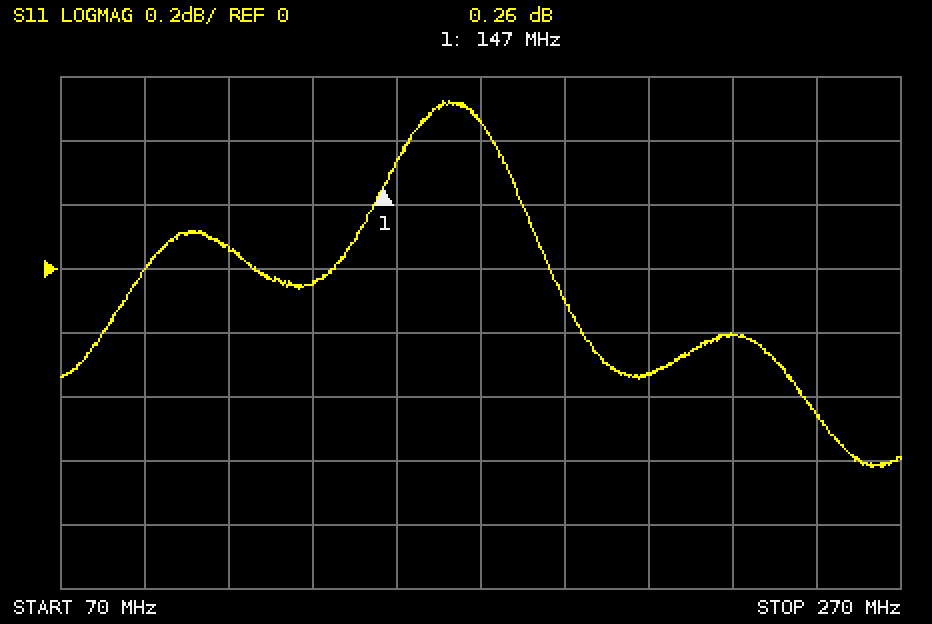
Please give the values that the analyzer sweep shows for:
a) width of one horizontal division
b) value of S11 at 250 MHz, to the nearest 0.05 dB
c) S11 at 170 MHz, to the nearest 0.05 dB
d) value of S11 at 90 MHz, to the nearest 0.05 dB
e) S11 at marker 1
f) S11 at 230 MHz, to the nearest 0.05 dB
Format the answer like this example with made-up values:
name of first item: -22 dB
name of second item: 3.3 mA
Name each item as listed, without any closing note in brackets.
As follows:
width of one horizontal division: 20 MHz
value of S11 at 250 MHz, to the nearest 0.05 dB: -0.45 dB
S11 at 170 MHz, to the nearest 0.05 dB: 0.45 dB
value of S11 at 90 MHz, to the nearest 0.05 dB: 0.00 dB
S11 at marker 1: 0.26 dB
S11 at 230 MHz, to the nearest 0.05 dB: -0.20 dB
